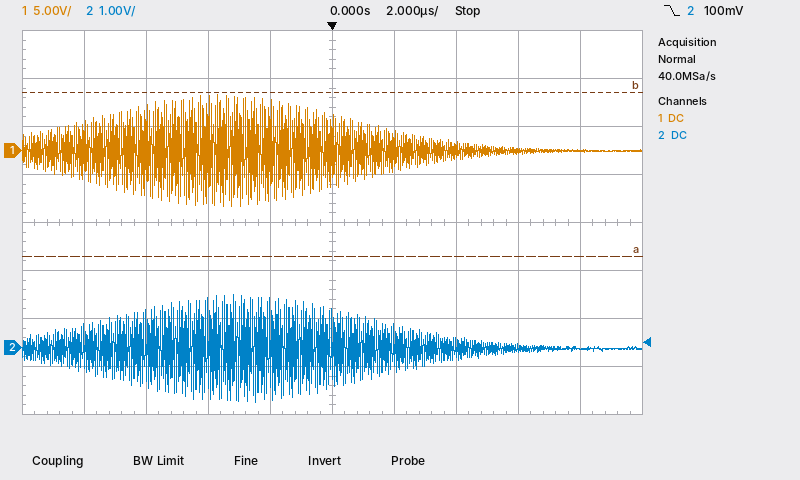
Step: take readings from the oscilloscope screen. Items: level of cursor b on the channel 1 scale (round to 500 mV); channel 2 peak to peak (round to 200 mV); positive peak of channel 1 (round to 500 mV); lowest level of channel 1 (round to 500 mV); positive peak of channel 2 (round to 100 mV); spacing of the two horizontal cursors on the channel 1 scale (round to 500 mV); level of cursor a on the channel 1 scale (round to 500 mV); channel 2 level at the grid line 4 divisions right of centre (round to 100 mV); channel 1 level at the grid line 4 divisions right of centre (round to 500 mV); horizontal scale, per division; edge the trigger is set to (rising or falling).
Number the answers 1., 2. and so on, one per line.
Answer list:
1. 6.0 V
2. 2.2 V
3. 6.0 V
4. -6.0 V
5. 1.1 V
6. 17.0 V
7. -11.0 V
8. 0.0 V
9. 0.0 V
10. 2 µs
11. falling
